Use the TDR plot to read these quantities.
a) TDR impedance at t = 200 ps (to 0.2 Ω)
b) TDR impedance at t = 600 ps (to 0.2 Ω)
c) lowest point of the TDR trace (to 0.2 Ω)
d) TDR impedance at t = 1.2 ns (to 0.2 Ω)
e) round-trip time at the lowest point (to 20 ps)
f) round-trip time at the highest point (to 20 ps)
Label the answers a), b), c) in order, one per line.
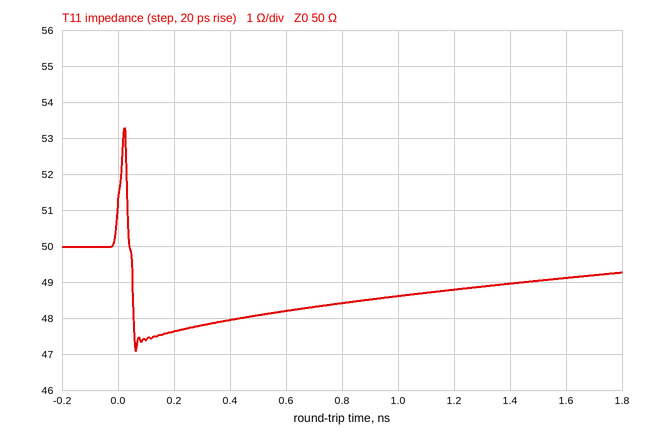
a) 47.6 Ω
b) 48.2 Ω
c) 47.0 Ω
d) 48.8 Ω
e) 60 ps
f) 20 ps
